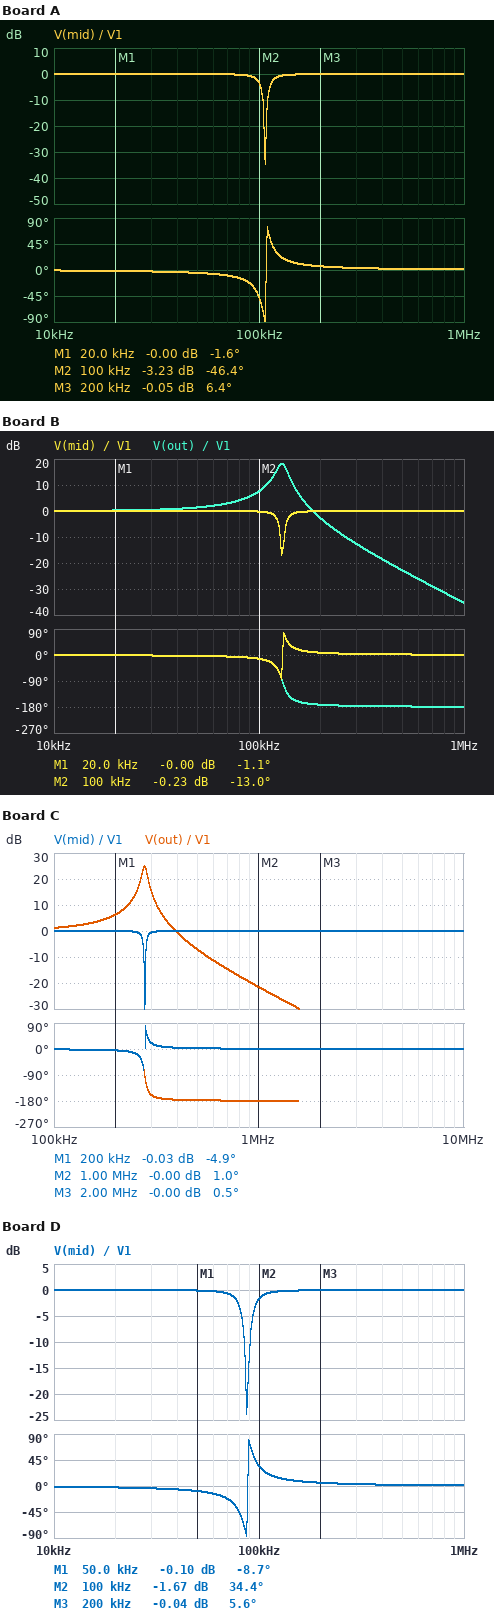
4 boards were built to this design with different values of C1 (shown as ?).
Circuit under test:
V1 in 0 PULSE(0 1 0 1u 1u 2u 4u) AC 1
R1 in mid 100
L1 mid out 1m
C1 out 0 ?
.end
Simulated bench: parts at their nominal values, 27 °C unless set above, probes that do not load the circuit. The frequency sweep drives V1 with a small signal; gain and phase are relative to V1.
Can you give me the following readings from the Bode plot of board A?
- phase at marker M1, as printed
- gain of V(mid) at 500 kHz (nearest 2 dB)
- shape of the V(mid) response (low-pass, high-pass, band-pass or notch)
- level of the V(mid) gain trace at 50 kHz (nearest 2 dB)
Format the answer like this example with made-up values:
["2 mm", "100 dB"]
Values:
["-1.6 deg", "0 dB", "notch", "0 dB"]
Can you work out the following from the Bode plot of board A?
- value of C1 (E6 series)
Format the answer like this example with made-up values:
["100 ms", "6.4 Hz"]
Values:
["2.2 nF"]
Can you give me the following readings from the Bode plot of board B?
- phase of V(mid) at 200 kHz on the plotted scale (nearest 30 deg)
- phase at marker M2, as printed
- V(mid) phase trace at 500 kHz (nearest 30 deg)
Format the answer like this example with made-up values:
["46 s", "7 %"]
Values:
["0 deg", "-13.0 deg", "0 deg"]
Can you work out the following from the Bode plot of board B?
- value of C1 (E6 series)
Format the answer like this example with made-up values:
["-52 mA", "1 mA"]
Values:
["1.5 nF"]
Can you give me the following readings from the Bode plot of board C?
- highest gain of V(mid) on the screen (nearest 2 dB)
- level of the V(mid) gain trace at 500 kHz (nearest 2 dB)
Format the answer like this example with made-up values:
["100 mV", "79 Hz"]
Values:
["0 dB", "0 dB"]
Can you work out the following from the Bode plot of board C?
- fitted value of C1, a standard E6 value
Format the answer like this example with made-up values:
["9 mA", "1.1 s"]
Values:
["330 pF"]
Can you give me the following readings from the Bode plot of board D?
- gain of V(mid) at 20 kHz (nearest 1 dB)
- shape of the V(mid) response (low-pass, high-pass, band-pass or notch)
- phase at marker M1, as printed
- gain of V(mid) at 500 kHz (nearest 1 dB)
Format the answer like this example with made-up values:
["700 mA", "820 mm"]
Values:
["0 dB", "notch", "-8.7 deg", "0 dB"]
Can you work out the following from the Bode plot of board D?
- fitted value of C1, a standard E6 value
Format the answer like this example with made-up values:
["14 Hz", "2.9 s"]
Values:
["3.3 nF"]
